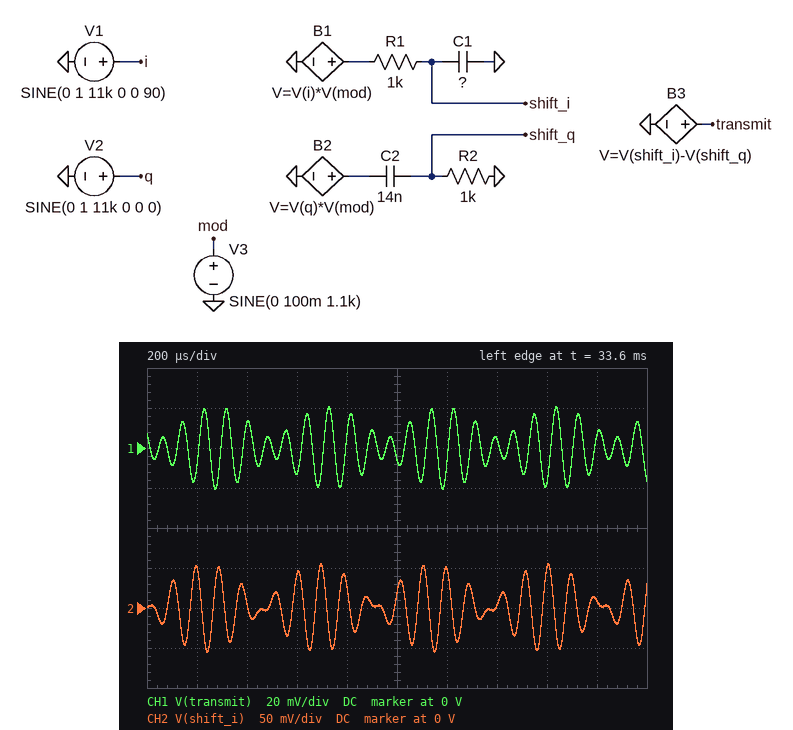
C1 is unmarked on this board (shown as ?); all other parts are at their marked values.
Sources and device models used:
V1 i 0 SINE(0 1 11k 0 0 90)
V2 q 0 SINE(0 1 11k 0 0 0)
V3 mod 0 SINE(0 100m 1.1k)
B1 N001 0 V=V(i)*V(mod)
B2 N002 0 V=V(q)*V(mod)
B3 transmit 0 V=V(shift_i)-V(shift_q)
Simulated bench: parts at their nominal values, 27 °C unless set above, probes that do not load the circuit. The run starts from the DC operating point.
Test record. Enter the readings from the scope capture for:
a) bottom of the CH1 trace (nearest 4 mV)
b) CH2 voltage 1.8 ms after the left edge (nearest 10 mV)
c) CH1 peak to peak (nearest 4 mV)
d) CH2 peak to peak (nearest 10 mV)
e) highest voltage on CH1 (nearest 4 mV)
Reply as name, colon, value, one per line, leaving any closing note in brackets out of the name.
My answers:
bottom of the CH1 trace: -20 mV
CH2 voltage 1.8 ms after the left edge: 10 mV
CH1 peak to peak: 40 mV
CH2 peak to peak: 110 mV
highest voltage on CH1: 20 mV
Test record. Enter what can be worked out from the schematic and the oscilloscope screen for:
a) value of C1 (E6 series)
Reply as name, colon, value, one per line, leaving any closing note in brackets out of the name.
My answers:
value of C1: 22 nF
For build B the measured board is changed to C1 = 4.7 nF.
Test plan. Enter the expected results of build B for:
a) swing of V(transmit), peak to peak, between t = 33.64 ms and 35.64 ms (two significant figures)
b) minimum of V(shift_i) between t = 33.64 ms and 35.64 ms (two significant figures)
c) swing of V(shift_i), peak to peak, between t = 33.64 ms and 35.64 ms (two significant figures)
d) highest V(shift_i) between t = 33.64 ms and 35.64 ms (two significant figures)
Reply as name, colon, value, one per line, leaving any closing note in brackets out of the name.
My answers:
swing of V(transmit), peak to peak, between t = 33.64 ms and 35.64 ms: 90 mV
minimum of V(shift_i) between t = 33.64 ms and 35.64 ms: -95 mV
swing of V(shift_i), peak to peak, between t = 33.64 ms and 35.64 ms: 190 mV
highest V(shift_i) between t = 33.64 ms and 35.64 ms: 95 mV
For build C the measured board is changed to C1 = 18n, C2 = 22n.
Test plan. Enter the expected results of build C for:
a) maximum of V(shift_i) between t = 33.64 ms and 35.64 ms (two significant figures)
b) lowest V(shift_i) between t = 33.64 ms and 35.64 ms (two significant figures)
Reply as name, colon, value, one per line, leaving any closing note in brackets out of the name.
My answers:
maximum of V(shift_i) between t = 33.64 ms and 35.64 ms: 63 mV
lowest V(shift_i) between t = 33.64 ms and 35.64 ms: -63 mV
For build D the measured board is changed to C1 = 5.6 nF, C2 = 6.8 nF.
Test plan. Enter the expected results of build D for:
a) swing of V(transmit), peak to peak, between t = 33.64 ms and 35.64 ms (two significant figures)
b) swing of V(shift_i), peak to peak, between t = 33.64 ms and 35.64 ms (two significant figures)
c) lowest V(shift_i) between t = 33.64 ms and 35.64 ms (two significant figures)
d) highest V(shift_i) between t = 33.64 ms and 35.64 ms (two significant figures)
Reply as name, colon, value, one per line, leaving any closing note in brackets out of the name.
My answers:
swing of V(transmit), peak to peak, between t = 33.64 ms and 35.64 ms: 100 mV
swing of V(shift_i), peak to peak, between t = 33.64 ms and 35.64 ms: 190 mV
lowest V(shift_i) between t = 33.64 ms and 35.64 ms: -93 mV
highest V(shift_i) between t = 33.64 ms and 35.64 ms: 93 mV
